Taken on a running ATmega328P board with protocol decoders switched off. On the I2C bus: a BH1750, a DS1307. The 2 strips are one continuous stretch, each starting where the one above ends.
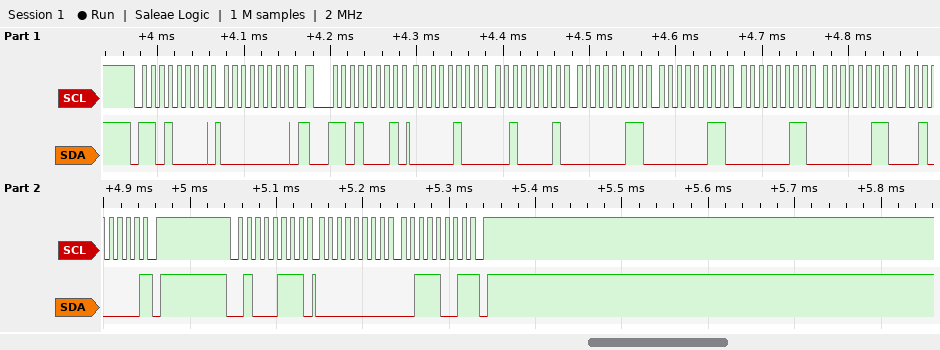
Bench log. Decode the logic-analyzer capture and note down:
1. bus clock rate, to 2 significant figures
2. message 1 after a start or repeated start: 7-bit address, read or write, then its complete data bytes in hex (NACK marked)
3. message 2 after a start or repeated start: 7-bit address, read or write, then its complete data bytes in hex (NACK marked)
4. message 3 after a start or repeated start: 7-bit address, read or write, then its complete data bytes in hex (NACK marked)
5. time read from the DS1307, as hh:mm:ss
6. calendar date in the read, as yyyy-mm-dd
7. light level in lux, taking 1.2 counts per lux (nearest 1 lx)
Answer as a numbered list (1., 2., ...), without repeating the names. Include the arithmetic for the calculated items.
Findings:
1. 100 kHz
2. 0x68 write: 00
3. 0x68 read: 04 21 03 03 03 03 20 NACK
4. 0x23 read: 00 39 NACK
5. 03:21:04
6. 2020-03-03
7. 57 / 1.2 = 48 lx
